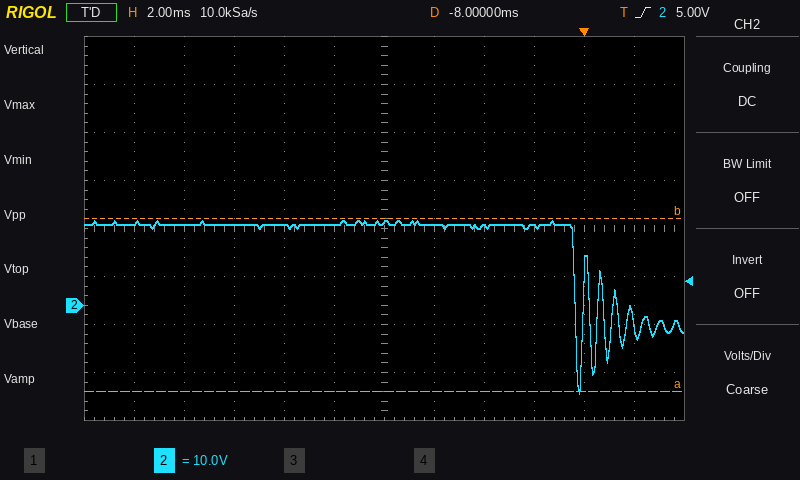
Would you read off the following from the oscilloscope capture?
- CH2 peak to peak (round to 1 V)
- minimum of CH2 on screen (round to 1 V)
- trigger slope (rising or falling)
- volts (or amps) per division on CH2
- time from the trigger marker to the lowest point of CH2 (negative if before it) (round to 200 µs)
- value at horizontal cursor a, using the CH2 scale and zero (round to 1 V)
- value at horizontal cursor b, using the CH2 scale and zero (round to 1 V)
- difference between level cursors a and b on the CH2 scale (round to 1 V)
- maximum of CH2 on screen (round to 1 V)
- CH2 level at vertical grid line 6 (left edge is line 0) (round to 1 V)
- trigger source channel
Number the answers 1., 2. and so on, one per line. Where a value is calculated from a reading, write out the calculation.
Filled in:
1. 18 V − (-18 V) = 36 V
2. -18 V
3. rising
4. 10 V
5. -200 µs
6. -18 V
7. 18 V
8. 36 V
9. 18 V
10. 17 V
11. CH2
